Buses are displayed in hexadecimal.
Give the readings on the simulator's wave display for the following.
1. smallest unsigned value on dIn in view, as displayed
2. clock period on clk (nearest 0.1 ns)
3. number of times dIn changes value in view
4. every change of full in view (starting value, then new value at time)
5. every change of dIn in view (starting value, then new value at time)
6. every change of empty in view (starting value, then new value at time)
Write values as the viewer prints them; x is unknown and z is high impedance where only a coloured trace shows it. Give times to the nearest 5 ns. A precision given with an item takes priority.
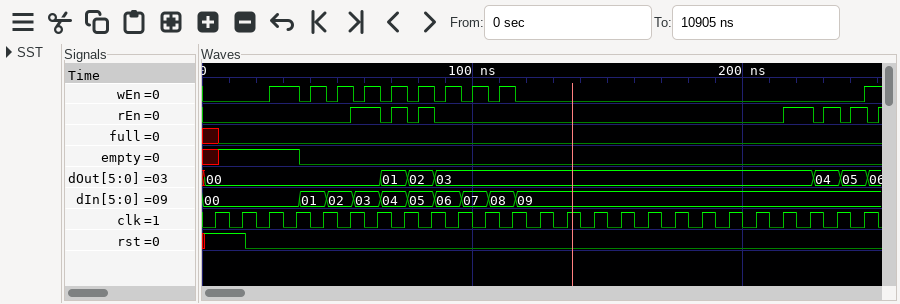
00
10 ns
9
x, 0 at 5 ns
00, 01 at 35 ns, 02 at 45 ns, 03 at 55 ns, 04 at 65 ns, 05 at 75 ns, 06 at 85 ns, 07 at 95 ns, 08 at 105 ns, 09 at 115 ns
x, 1 at 5 ns, 0 at 35 ns
